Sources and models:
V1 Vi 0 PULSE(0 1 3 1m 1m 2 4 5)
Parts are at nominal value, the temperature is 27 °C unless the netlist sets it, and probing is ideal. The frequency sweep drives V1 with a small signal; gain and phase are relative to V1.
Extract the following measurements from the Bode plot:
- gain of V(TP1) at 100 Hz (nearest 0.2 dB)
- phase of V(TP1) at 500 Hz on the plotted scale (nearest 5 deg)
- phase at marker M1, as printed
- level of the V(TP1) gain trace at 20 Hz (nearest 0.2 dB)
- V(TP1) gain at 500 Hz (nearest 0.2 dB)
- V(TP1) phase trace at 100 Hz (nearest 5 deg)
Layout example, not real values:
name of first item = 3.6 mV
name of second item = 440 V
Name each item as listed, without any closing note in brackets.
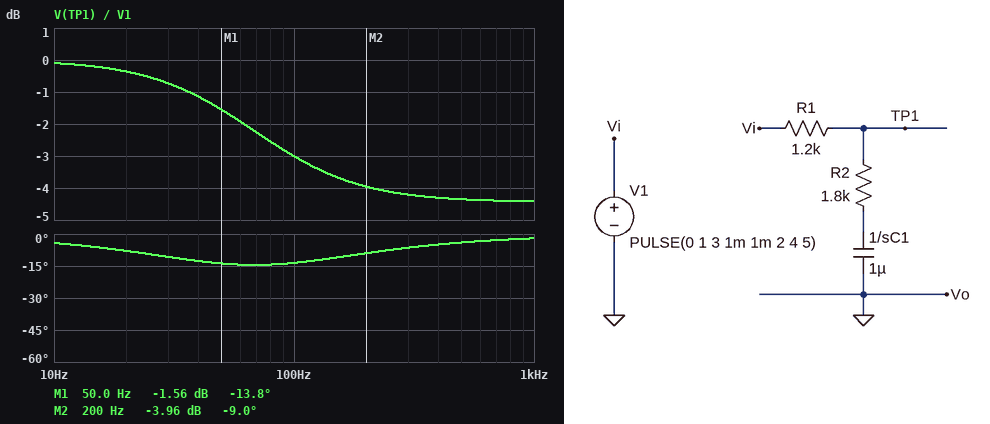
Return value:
gain of V(TP1) at 100 Hz = -3.0 dB
phase of V(TP1) at 500 Hz on the plotted scale = -5 deg
phase at marker M1, as printed = -13.8 deg
level of the V(TP1) gain trace at 20 Hz = -0.4 dB
V(TP1) gain at 500 Hz = -4.4 dB
V(TP1) phase trace at 100 Hz = -15 deg
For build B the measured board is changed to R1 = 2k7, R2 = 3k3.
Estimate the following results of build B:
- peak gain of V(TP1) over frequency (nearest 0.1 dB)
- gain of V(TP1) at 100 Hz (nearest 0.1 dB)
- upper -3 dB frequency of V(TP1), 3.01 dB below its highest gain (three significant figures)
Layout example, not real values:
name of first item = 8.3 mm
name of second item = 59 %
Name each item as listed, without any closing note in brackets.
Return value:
peak gain of V(TP1) over frequency = 0 dB
gain of V(TP1) at 100 Hz = -4.6 dB
upper -3 dB frequency of V(TP1), 3.01 dB below its highest gain = 42.2 Hz
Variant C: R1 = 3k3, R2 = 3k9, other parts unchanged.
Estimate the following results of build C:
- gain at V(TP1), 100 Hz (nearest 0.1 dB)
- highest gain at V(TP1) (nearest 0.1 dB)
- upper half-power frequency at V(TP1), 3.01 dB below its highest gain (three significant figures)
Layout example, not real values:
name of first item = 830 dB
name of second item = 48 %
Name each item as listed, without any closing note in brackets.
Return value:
gain at V(TP1), 100 Hz = -4.9 dB
highest gain at V(TP1) = 0 dB
upper half-power frequency at V(TP1), 3.01 dB below its highest gain = 34.4 Hz
